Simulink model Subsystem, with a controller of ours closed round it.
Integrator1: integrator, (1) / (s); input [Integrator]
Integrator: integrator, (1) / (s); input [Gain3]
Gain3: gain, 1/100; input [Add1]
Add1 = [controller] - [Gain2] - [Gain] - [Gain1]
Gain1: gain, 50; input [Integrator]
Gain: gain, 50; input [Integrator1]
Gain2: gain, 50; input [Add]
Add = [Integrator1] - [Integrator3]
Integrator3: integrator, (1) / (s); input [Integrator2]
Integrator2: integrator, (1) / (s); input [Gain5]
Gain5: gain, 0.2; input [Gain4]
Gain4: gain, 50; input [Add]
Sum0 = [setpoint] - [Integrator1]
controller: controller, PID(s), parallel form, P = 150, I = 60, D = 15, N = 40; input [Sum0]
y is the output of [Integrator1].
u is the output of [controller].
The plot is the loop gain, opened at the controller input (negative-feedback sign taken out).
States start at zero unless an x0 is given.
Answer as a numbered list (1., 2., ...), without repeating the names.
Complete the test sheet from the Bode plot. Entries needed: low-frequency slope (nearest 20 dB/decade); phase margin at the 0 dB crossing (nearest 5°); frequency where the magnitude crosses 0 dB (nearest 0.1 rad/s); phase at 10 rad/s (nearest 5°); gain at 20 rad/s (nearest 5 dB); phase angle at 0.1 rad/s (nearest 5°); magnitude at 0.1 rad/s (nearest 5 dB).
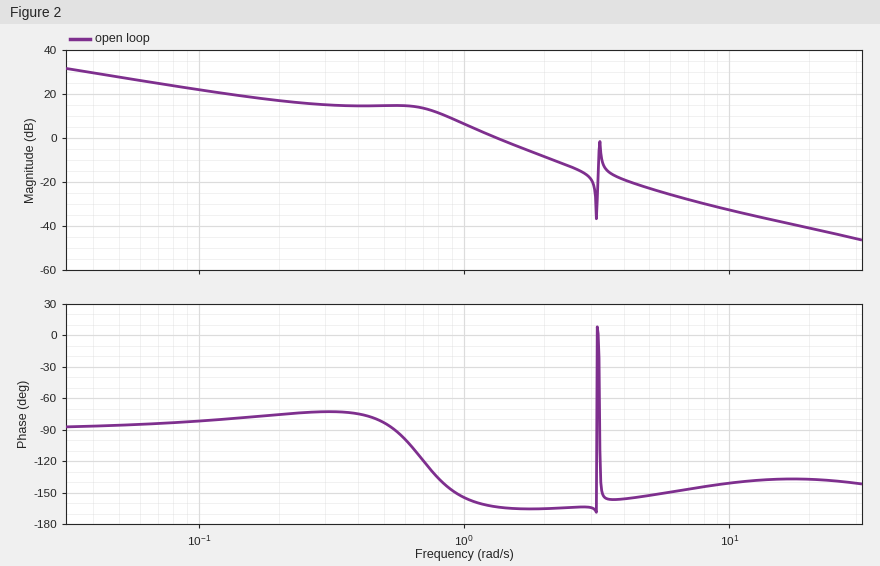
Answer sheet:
1. -20 dB/decade
2. 15°
3. 1.3 rad/s
4. -140°
5. -40 dB
6. -80°
7. 20 dB
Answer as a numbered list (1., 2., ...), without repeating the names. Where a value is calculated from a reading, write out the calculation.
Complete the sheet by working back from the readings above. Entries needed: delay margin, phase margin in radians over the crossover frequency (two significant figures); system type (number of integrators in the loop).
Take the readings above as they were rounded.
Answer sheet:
1. 15 × π / 180 / 1.3 = 0.20 s
2. 1
